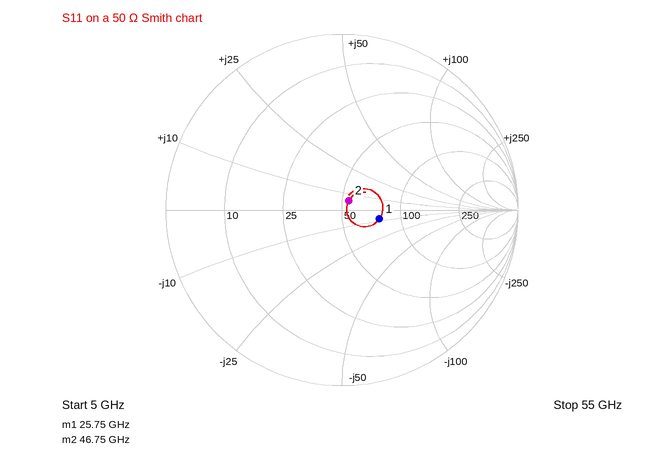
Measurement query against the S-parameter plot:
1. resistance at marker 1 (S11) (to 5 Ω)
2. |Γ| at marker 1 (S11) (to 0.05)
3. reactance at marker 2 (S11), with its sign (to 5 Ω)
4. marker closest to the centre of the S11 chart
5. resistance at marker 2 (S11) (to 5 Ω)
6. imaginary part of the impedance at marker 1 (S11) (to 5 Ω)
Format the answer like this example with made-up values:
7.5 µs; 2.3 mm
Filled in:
75 Ω; 0.20; +5 Ω; marker 2; 55 Ω; -10 Ω
